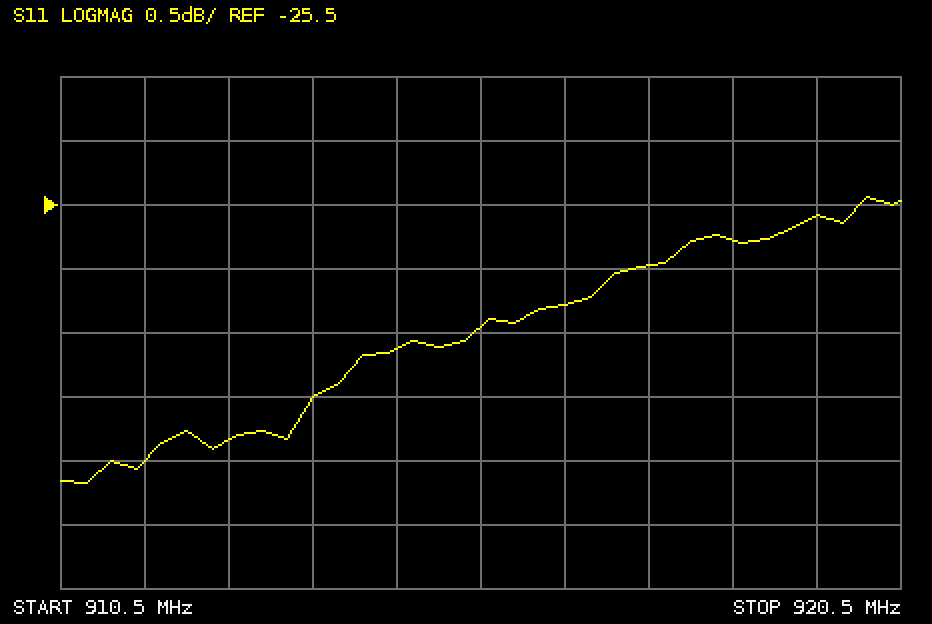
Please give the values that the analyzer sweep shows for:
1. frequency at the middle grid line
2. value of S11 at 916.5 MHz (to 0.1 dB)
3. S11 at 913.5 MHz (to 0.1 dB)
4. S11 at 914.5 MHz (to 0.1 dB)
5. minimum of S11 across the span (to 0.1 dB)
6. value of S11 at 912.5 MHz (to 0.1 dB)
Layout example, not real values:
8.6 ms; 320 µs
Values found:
915.5 MHz; -26.3 dB; -27.0 dB; -26.6 dB; -27.7 dB; -27.3 dB
